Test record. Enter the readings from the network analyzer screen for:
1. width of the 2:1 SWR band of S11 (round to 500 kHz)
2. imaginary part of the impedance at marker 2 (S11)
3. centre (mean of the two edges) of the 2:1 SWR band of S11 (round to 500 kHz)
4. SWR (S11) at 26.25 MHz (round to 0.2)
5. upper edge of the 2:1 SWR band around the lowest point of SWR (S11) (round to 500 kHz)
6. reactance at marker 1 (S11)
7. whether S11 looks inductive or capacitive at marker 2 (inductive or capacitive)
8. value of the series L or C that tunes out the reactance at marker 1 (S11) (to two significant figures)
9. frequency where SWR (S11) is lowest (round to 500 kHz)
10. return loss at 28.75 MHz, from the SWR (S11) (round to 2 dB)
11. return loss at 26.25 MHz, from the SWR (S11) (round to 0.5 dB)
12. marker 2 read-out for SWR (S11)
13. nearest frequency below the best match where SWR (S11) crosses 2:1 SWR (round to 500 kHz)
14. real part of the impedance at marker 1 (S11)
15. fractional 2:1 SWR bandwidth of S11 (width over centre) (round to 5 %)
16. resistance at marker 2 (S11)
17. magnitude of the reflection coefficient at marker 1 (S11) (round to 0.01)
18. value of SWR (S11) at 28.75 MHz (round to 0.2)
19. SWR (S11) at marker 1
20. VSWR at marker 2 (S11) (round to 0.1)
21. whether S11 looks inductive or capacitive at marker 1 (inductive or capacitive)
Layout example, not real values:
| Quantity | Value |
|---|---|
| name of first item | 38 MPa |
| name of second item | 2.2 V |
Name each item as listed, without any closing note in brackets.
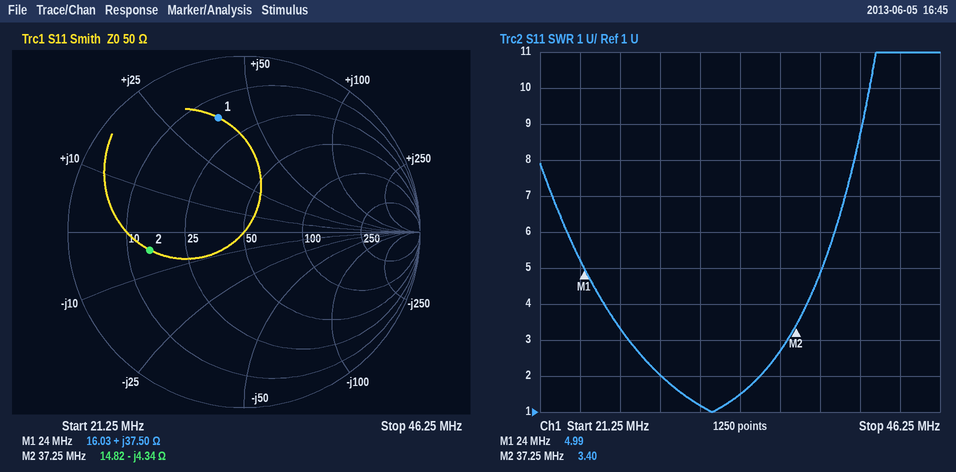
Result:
| Quantity | Value |
|---|---|
| width of the 2:1 SWR band of S11 | 6.0 MHz |
| imaginary part of the impedance at marker 2 | -4.34 Ω |
| centre (mean of the two edges) of the 2:1 SWR band of S11 | 32.0 MHz |
| SWR (S11) at 26.25 MHz | 3.4 |
| upper edge of the 2:1 SWR band around the lowest point of SWR (S11) | 35.0 MHz |
| reactance at marker 1 | +37.50 Ω |
| whether S11 looks inductive or capacitive at marker 2 | capacitive |
| value of the series L or C that tunes out the reactance at marker 1 (S11) | 180 pF |
| frequency where SWR (S11) is lowest | 32.0 MHz |
| return loss at 28.75 MHz, from the SWR (S11) | 10 dB |
| return loss at 26.25 MHz, from the SWR (S11) | 5.5 dB |
| marker 2 read-out for SWR | 3.40 |
| nearest frequency below the best match where SWR (S11) crosses 2:1 SWR | 29.0 MHz |
| real part of the impedance at marker 1 | 16.03 Ω |
| fractional 2:1 SWR bandwidth of S11 (width over centre) | 20 % |
| resistance at marker 2 | 14.82 Ω |
| magnitude of the reflection coefficient at marker 1 (S11) | 0.67 |
| value of SWR (S11) at 28.75 MHz | 2.0 |
| SWR (S11) at marker 1 | 4.99 |
| VSWR at marker 2 (S11) | 3.4 |
| whether S11 looks inductive or capacitive at marker 1 | inductive |
